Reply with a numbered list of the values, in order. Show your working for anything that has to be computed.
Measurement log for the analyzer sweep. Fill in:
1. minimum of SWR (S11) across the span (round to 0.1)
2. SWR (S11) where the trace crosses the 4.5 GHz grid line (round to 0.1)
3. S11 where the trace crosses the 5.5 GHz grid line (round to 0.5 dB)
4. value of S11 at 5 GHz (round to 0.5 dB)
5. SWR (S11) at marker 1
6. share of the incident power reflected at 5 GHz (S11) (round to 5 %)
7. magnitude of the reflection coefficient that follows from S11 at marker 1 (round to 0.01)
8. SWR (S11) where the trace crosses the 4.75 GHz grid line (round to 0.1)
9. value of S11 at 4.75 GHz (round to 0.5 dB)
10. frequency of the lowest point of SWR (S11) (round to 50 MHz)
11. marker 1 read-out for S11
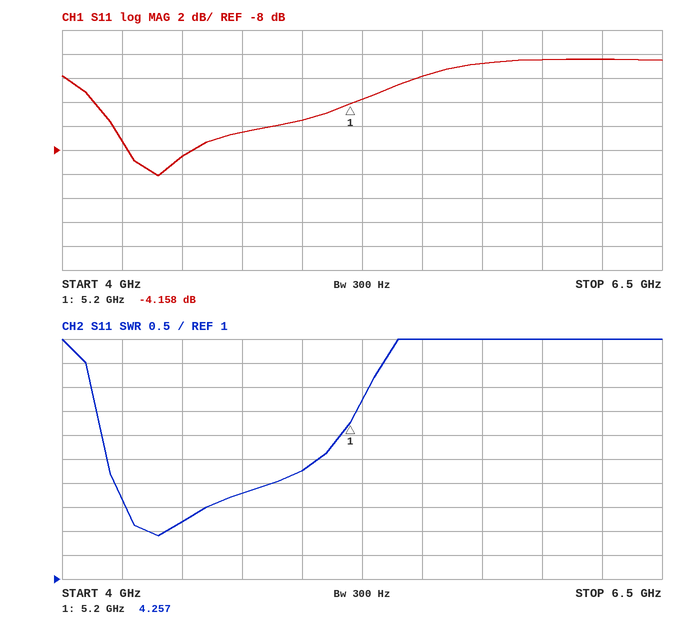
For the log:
1. 1.9
2. 2.2
3. -2.0 dB
4. -5.5 dB
5. 4.257
6. 10^(-5.5/10) ≈ 28.2 %, so 30 % to the nearest 5 %
7. 10^(-4.158/20) ≈ 0.62
8. 2.8
9. -6.5 dB
10. 4.40 GHz
11. -4.158 dB
